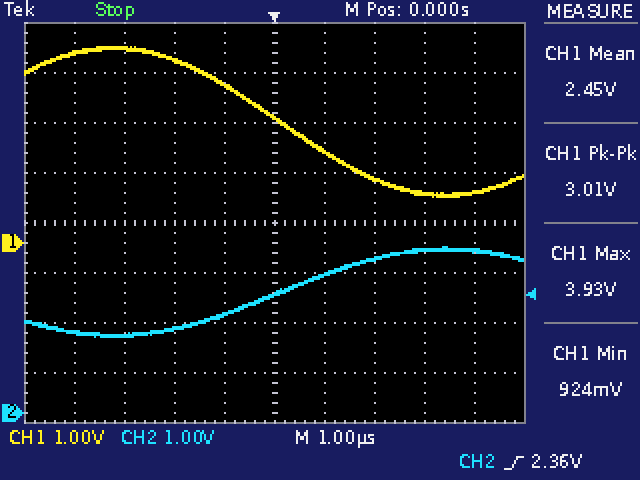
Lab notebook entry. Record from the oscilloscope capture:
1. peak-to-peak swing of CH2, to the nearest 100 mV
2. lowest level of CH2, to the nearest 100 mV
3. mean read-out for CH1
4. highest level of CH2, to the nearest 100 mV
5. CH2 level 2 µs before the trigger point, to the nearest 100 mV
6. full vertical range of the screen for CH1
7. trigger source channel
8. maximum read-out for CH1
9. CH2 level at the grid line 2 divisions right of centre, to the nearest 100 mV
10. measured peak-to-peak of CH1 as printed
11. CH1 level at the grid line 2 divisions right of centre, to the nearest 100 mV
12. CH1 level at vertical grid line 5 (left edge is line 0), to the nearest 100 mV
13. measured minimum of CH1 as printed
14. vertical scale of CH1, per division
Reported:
1.8 V
1.5 V
2.45 V
3.3 V
1.7 V
8 V
CH2
3.93 V
3.1 V
3.01 V
1.3 V
2.5 V
924 mV
1 V
